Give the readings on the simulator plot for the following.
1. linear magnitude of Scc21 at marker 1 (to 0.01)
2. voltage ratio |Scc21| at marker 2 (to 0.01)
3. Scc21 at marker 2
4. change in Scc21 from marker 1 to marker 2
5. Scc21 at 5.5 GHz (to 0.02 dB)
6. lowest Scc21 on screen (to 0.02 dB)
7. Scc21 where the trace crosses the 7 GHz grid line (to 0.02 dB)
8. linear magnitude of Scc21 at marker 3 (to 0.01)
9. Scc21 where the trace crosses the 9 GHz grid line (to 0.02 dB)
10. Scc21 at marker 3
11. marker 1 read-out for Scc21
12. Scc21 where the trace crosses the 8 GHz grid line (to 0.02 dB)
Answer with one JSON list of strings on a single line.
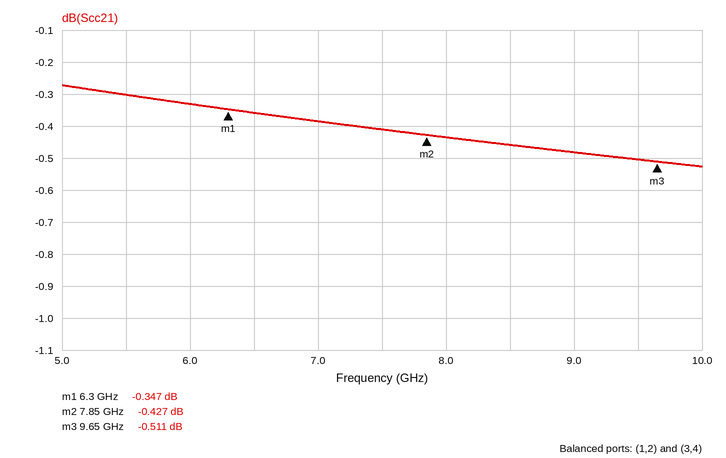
["0.96", "0.95", "-0.427 dB", "-0.080 dB", "-0.30 dB", "-0.52 dB", "-0.38 dB", "0.94", "-0.48 dB", "-0.511 dB", "-0.347 dB", "-0.44 dB"]
